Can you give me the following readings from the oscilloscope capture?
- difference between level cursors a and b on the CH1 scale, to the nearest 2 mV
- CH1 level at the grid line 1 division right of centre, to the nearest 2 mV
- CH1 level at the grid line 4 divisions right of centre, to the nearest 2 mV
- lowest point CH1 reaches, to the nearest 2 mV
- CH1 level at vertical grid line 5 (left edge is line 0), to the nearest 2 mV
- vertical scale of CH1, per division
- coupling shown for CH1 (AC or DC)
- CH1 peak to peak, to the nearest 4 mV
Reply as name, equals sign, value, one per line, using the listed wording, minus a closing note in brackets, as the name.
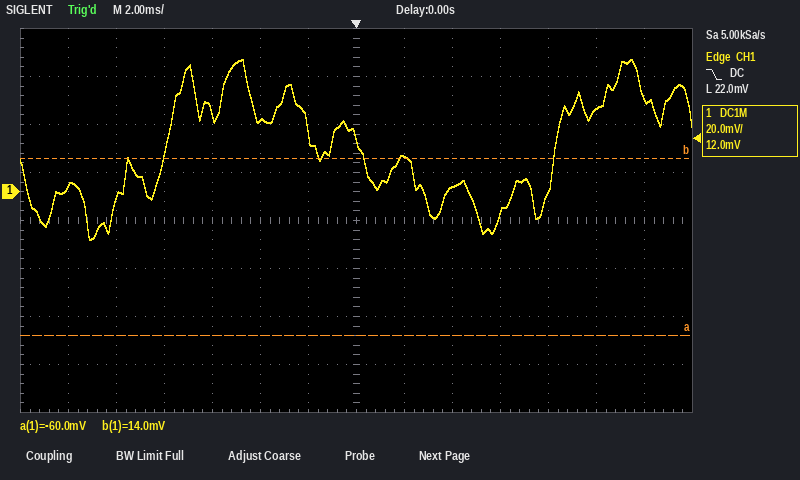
difference between level cursors a and b on the CH1 scale, to the nearest 2 mV = 74 mV
CH1 level at the grid line 1 division right of centre, to the nearest 2 mV = 14 mV
CH1 level at the grid line 4 divisions right of centre, to the nearest 2 mV = 0 mV
lowest point CH1 reaches, to the nearest 2 mV = -20 mV
CH1 level at vertical grid line 5 (left edge is line 0), to the nearest 2 mV = 30 mV
vertical scale of CH1, per division = 20 mV
coupling shown for CH1 = DC
CH1 peak to peak, to the nearest 4 mV = 76 mV
